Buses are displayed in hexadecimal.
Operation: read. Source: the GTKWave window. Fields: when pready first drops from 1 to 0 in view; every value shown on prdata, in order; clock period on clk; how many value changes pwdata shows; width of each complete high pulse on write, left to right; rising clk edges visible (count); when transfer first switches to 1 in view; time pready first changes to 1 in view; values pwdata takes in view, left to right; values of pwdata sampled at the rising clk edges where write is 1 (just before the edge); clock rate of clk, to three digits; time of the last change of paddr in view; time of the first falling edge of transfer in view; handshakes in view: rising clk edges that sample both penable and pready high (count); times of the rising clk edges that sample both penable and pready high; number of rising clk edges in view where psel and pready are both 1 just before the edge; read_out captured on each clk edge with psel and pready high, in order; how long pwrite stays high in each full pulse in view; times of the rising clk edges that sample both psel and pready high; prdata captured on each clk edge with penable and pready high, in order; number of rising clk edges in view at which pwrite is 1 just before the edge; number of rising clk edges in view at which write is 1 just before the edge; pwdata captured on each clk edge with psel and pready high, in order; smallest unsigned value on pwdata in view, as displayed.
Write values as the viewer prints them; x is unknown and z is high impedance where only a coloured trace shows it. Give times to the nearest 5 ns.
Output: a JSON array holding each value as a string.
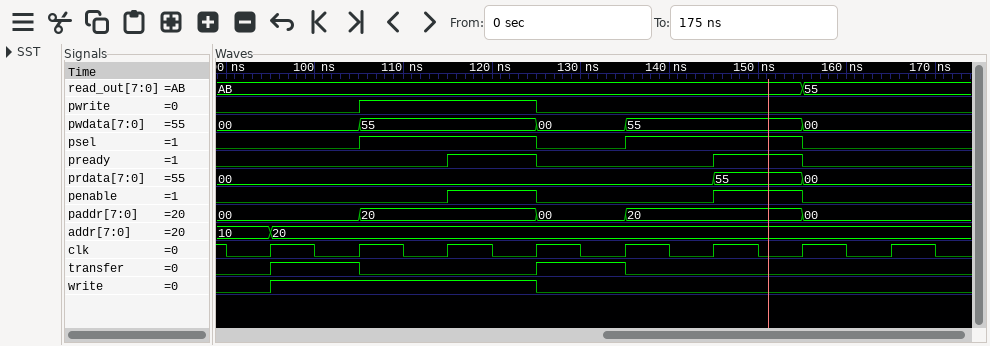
["125 ns", "00, 55, 00", "10 ns", "4", "30 ns", "8", "95 ns", "115 ns", "00, 55, 00, 55, 00", "00, 55, 55", "100 MHz", "155 ns", "105 ns", "2", "125 ns, 155 ns", "2", "AB, AB", "20 ns", "125 ns, 155 ns", "00, 55", "2", "3", "55, 55", "00"]
